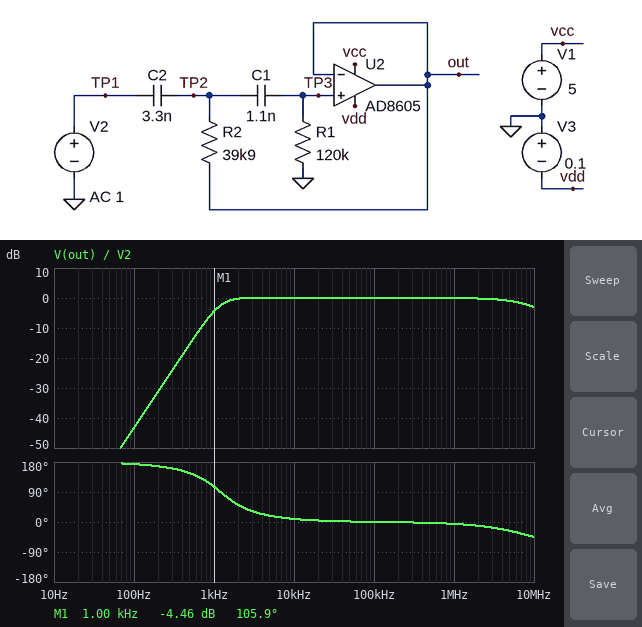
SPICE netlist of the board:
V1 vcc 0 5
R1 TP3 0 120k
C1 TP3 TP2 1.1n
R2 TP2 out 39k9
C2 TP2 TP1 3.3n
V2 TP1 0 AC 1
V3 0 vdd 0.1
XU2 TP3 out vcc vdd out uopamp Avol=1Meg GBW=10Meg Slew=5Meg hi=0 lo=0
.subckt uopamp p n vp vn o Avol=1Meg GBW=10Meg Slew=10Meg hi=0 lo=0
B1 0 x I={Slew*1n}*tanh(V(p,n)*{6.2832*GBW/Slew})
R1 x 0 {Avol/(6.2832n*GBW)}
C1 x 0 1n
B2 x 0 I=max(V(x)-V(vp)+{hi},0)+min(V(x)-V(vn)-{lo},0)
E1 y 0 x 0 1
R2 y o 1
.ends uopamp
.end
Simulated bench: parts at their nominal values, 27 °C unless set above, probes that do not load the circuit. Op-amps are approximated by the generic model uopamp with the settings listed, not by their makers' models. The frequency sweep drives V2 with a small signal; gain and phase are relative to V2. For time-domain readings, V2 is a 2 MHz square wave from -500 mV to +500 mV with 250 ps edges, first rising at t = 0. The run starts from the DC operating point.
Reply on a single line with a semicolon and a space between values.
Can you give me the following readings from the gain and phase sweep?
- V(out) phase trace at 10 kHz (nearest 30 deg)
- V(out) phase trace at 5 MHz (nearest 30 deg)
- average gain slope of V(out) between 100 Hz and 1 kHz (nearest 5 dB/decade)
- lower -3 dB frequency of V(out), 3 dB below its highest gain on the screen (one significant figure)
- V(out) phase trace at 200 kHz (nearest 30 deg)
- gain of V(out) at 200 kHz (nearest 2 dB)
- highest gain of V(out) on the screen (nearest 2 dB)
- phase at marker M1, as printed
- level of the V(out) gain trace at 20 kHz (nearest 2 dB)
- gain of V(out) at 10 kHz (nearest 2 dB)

0 deg; -30 deg; 40 dB/decade; 1 kHz; 0 deg; 0 dB; 0 dB; 105.9 deg; 0 dB; 0 dB
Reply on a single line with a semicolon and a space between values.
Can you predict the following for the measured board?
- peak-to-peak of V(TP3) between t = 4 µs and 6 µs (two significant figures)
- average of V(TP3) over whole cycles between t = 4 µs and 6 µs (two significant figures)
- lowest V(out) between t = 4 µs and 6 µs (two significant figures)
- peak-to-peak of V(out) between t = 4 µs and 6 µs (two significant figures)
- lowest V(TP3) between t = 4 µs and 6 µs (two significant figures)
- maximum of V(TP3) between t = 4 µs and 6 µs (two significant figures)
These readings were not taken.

1.0 V; 470 mV; -28 mV; 1.0 V; -31 mV; 980 mV
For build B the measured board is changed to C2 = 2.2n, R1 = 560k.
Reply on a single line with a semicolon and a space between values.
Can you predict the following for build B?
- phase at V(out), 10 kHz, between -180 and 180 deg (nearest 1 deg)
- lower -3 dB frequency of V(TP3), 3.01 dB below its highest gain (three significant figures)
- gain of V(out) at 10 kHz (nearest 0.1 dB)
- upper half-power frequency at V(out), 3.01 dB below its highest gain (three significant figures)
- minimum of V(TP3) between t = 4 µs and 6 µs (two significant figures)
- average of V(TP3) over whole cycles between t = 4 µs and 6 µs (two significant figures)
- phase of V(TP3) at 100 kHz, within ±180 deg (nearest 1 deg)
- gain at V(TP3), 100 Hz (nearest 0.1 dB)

2 deg; 582 Hz; 0 dB; 1.26 kHz; -8.5 mV; 490 mV; 0 deg; -33.3 dB
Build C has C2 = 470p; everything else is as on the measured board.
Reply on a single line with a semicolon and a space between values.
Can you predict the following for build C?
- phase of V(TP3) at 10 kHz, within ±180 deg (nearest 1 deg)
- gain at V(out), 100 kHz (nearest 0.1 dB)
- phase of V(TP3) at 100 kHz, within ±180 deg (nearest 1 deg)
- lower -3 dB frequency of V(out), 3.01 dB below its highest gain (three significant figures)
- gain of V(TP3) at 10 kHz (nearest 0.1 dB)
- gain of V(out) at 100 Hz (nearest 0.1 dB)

24 deg; 0 dB; 2 deg; 2.94 kHz; 0.1 dB; -60.2 dB
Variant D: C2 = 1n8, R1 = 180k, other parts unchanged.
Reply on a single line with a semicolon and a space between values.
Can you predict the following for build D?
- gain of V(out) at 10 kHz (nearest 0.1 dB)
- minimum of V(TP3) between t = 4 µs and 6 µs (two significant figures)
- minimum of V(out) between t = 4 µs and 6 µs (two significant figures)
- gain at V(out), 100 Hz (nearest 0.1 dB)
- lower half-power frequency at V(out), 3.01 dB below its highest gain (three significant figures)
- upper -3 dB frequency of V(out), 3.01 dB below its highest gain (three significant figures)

0.1 dB; -26 mV; -23 mV; -45.0 dB; 1.14 kHz; 6.63 MHz
